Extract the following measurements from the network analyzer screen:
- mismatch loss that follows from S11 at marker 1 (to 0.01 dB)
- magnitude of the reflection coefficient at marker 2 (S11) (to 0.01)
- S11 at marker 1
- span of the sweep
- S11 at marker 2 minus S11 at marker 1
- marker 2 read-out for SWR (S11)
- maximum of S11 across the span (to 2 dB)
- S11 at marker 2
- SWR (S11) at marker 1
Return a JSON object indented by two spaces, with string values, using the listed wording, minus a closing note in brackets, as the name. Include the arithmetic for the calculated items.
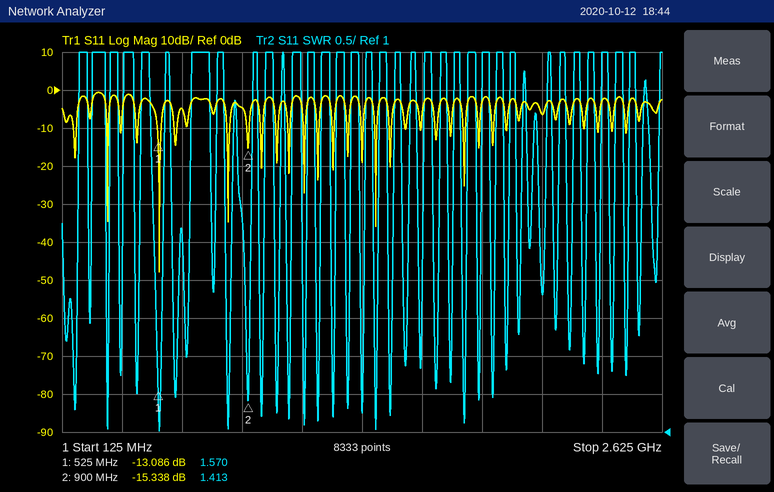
{
  "mismatch loss that follows from S11 at marker 1": "−10 log10(1 − 10^(-13.086/10)) ≈ 0.22 dB",
  "magnitude of the reflection coefficient at marker 2 (S11)": "10^(-15.338/20) ≈ 0.17",
  "S11 at marker 1": "-13.086 dB",
  "span of the sweep": "2.5 GHz",
  "S11 at marker 2 minus S11 at marker 1": "-15.338 − (-13.086) = -2.252 dB",
  "marker 2 read-out for SWR": "1.413",
  "maximum of S11 across the span": "0 dB",
  "S11 at marker 2": "-15.338 dB",
  "SWR (S11) at marker 1": "1.570"
}
